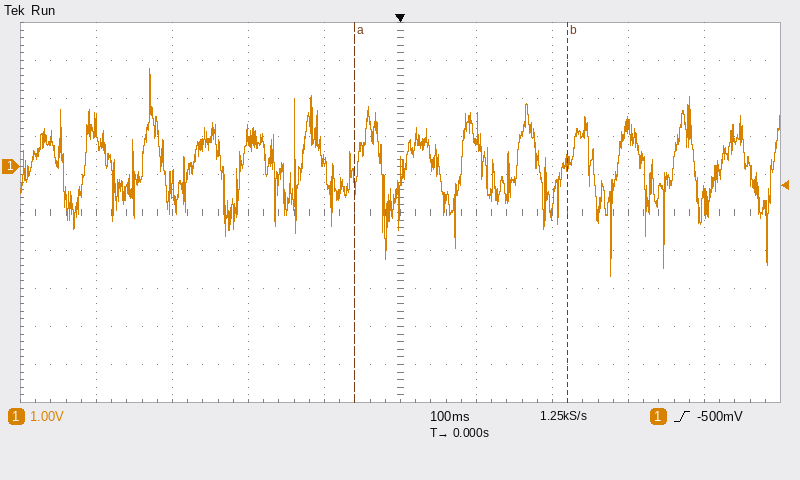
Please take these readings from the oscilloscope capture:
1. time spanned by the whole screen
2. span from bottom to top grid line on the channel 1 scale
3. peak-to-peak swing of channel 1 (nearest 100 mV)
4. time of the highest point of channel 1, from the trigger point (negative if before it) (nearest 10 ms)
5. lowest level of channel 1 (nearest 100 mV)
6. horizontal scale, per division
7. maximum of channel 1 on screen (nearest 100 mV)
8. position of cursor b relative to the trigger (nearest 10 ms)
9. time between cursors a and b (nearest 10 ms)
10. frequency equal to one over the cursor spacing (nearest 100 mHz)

1 s
10 V
5.5 V
-330 ms
-2.9 V
100 ms
2.6 V
+220 ms
280 ms
3.6 Hz
